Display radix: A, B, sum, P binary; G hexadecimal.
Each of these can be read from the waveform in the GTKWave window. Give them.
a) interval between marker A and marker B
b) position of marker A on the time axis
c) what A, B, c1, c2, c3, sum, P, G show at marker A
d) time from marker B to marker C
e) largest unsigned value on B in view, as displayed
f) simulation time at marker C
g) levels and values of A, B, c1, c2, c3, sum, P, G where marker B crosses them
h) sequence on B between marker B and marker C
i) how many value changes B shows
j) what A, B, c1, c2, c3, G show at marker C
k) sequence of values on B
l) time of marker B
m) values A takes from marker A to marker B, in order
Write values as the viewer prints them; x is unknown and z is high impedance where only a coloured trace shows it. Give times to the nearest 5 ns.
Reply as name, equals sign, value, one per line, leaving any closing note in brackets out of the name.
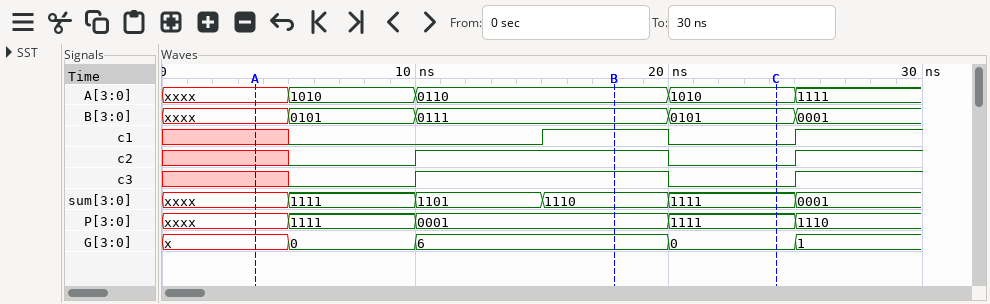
interval between marker A and marker B = 15 ns
position of marker A on the time axis = 5 ns
what A, B, c1, c2, c3, sum, P, G show at marker A = A=xxxx, B=xxxx, c1=x, c2=x, c3=x, sum=xxxx, P=xxxx, G=x
time from marker B to marker C = 5 ns
largest unsigned value on B in view, as displayed = 0111
simulation time at marker C = 25 ns
levels and values of A, B, c1, c2, c3, sum, P, G where marker B crosses them = A=0110, B=0111, c1=1, c2=1, c3=1, sum=1110, P=0001, G=6
sequence on B between marker B and marker C = 0111, 0101
how many value changes B shows = 4
what A, B, c1, c2, c3, G show at marker C = A=1010, B=0101, c1=0, c2=0, c3=0, G=0
sequence of values on B = xxxx, 0101, 0111, 0101, 0001
time of marker B = 20 ns
values A takes from marker A to marker B, in order = xxxx, 1010, 0110
